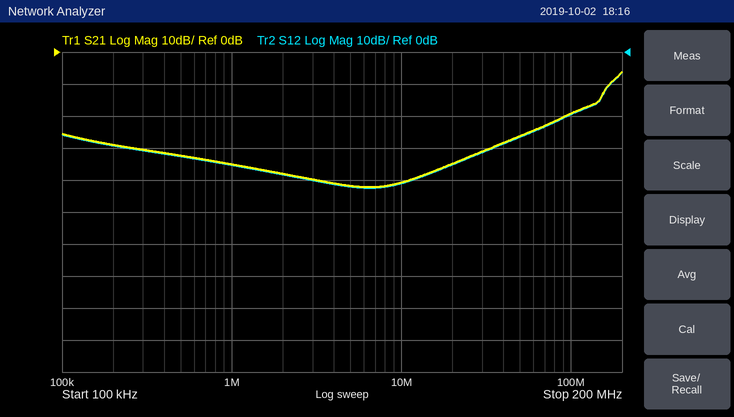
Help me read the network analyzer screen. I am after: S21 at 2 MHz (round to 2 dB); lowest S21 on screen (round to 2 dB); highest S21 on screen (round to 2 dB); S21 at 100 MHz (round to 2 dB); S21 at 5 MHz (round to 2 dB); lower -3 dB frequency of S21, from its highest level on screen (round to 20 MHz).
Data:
-38 dB
-42 dB
-6 dB
-20 dB
-42 dB
180 MHz
